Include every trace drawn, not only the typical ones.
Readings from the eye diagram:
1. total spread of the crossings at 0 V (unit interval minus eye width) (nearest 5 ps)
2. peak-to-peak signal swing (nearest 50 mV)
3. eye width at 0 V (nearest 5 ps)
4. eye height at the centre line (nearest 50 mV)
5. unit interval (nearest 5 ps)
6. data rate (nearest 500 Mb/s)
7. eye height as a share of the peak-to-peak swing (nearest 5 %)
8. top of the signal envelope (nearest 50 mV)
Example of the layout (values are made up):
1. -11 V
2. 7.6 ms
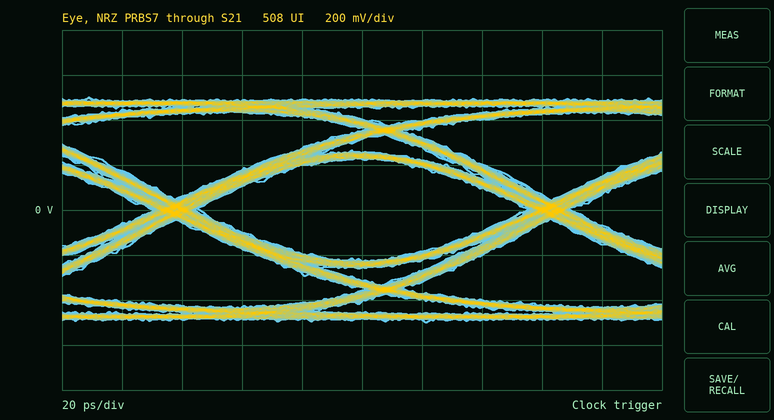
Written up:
1. 15 ps
2. 1.00 V
3. 110 ps
4. 450 mV
5. 125 ps
6. 8.0 Gb/s
7. 45 %
8. 500 mV
